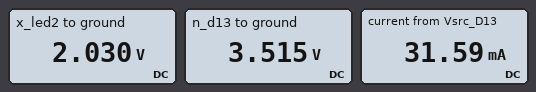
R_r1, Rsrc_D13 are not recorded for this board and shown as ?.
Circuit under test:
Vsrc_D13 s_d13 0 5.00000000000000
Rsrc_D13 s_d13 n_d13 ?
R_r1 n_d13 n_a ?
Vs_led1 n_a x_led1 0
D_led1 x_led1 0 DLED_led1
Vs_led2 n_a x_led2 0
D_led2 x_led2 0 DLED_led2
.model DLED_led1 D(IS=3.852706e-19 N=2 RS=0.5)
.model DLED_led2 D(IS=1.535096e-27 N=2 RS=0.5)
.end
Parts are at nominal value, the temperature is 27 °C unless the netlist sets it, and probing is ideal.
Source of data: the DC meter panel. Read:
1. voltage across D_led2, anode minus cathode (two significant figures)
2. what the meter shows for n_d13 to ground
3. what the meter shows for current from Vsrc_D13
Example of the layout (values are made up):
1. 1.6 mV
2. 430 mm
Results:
1. 2.0 V
2. 3.515 V
3. 31.59 mA
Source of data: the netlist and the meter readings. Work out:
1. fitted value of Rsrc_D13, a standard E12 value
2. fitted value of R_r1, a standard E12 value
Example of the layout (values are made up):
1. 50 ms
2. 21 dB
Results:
1. 47 Ω
2. 47 Ω
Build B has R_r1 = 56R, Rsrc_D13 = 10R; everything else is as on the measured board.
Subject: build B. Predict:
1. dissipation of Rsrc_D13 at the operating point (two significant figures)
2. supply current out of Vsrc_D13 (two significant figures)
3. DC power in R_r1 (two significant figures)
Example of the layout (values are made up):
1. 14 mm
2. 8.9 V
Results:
1. 20 mW
2. 45 mA
3. 110 mW
